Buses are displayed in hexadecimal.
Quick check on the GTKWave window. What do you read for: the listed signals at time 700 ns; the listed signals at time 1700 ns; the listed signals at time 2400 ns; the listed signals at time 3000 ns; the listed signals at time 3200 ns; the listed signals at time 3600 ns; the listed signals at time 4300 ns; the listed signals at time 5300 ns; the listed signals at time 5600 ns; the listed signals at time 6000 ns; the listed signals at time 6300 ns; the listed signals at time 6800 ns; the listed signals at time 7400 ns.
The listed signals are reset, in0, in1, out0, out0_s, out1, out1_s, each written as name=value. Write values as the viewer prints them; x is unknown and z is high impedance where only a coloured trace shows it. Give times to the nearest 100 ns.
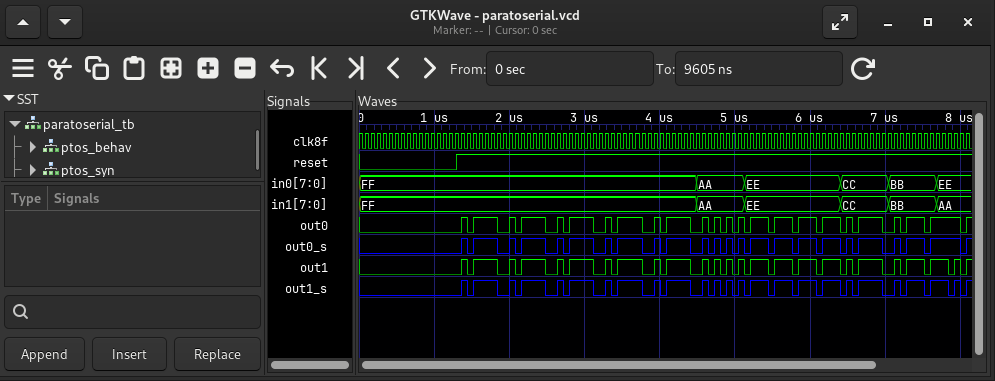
reset=0, in0=FF, in1=FF, out0=0, out0_s=0, out1=0, out1_s=0
reset=1, in0=FF, in1=FF, out0=1, out0_s=1, out1=1, out1_s=1
reset=1, in0=FF, in1=FF, out0=1, out0_s=1, out1=1, out1_s=1
reset=1, in0=FF, in1=FF, out0=1, out0_s=1, out1=1, out1_s=1
reset=1, in0=FF, in1=FF, out0=0, out0_s=0, out1=0, out1_s=0
reset=1, in0=FF, in1=FF, out0=1, out0_s=1, out1=1, out1_s=1
reset=1, in0=FF, in1=FF, out0=1, out0_s=1, out1=1, out1_s=1
reset=1, in0=EE, in1=EE, out0=1, out0_s=1, out1=1, out1_s=1
reset=1, in0=EE, in1=EE, out0=1, out0_s=1, out1=1, out1_s=1
reset=1, in0=EE, in1=EE, out0=1, out0_s=1, out1=1, out1_s=1
reset=1, in0=EE, in1=EE, out0=1, out0_s=1, out1=1, out1_s=1
reset=1, in0=CC, in1=CC, out0=1, out0_s=1, out1=1, out1_s=1
reset=1, in0=BB, in1=BB, out0=1, out0_s=1, out1=1, out1_s=1
